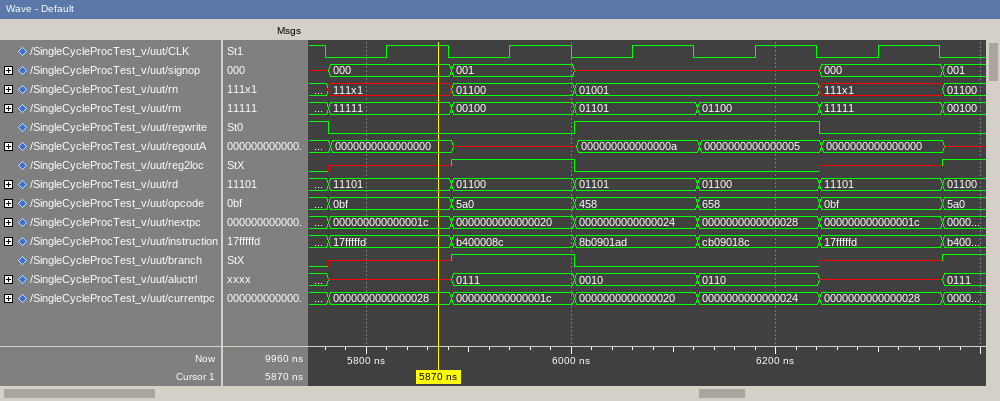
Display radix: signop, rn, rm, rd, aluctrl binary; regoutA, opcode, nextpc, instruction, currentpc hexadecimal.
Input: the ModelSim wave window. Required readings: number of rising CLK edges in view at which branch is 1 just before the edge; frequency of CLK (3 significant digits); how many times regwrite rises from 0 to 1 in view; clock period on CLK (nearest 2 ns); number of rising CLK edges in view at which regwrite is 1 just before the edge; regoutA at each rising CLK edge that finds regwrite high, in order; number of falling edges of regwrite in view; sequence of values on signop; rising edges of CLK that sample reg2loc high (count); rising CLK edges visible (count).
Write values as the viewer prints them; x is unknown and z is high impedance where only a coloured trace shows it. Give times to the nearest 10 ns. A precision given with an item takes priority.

1
8.33 MHz
1
120 ns
2
000000000000000a, 0000000000000005
2
x, 000, 001, x, 000, 001
1
5
